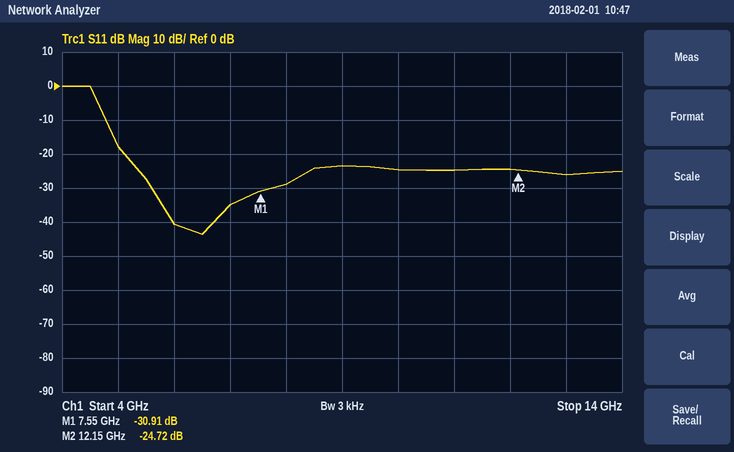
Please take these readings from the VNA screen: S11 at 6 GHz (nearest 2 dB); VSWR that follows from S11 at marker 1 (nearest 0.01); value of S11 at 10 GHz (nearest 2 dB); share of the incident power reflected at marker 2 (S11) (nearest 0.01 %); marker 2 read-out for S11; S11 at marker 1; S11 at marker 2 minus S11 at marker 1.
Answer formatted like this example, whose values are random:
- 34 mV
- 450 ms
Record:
- -40 dB
- 1.06
- -24 dB
- 0.34 %
- -24.72 dB
- -30.91 dB
- 6.19 dB
